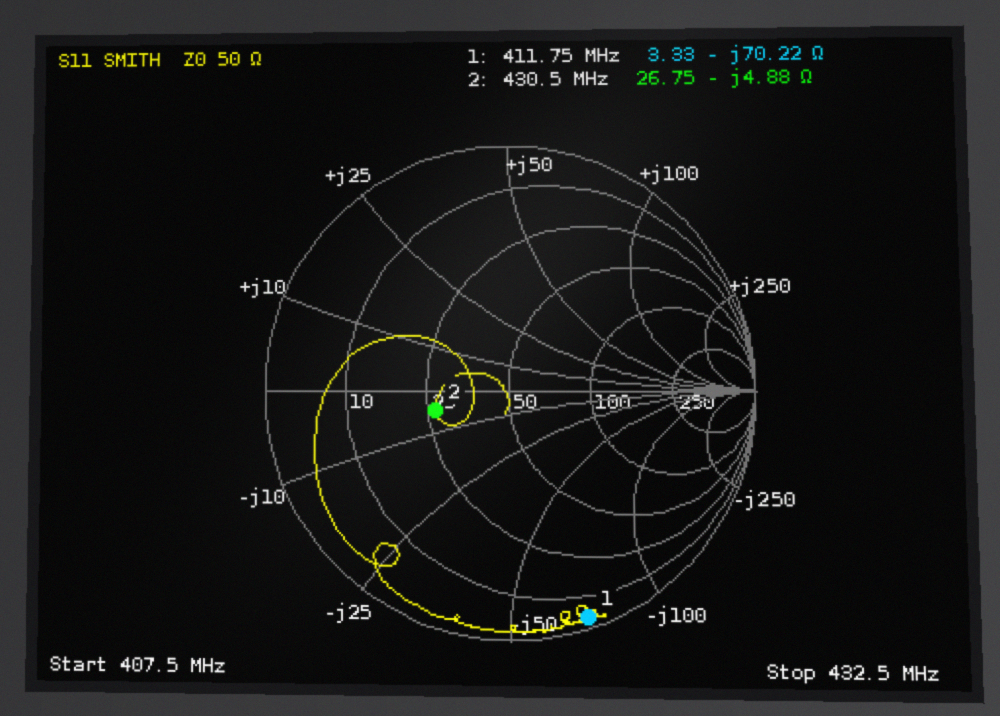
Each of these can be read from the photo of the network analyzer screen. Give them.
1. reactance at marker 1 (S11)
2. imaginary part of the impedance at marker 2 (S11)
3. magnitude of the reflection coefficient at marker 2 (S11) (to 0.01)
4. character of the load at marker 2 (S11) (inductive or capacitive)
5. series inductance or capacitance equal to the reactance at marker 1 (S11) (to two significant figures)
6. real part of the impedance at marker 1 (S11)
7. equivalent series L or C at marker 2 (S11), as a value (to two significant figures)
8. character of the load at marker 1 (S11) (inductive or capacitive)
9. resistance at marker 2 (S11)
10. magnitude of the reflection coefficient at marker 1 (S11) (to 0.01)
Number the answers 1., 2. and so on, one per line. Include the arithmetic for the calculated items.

1. -70.22 Ω
2. -4.88 Ω
3. 0.31
4. capacitive
5. C = 1/(2π × 411.75 MHz × 70.22 Ω) ≈ 5.5 pF
6. 3.33 Ω
7. C = 1/(2π × 430.5 MHz × 4.88 Ω) ≈ 76 pF
8. capacitive
9. 26.75 Ω
10. 0.96
